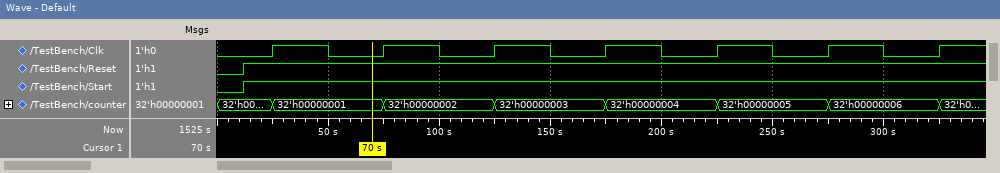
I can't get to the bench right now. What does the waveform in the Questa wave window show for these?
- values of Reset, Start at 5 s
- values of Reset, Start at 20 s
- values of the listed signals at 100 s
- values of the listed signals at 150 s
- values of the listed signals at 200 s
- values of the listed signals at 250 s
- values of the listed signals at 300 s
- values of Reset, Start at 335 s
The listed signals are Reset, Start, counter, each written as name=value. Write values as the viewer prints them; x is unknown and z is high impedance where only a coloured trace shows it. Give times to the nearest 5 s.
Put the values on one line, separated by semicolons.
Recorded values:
Reset=0, Start=0; Reset=1, Start=1; Reset=1, Start=1, counter=32'h00000002; Reset=1, Start=1, counter=32'h00000003; Reset=1, Start=1, counter=32'h00000004; Reset=1, Start=1, counter=32'h00000005; Reset=1, Start=1, counter=32'h00000006; Reset=1, Start=1
